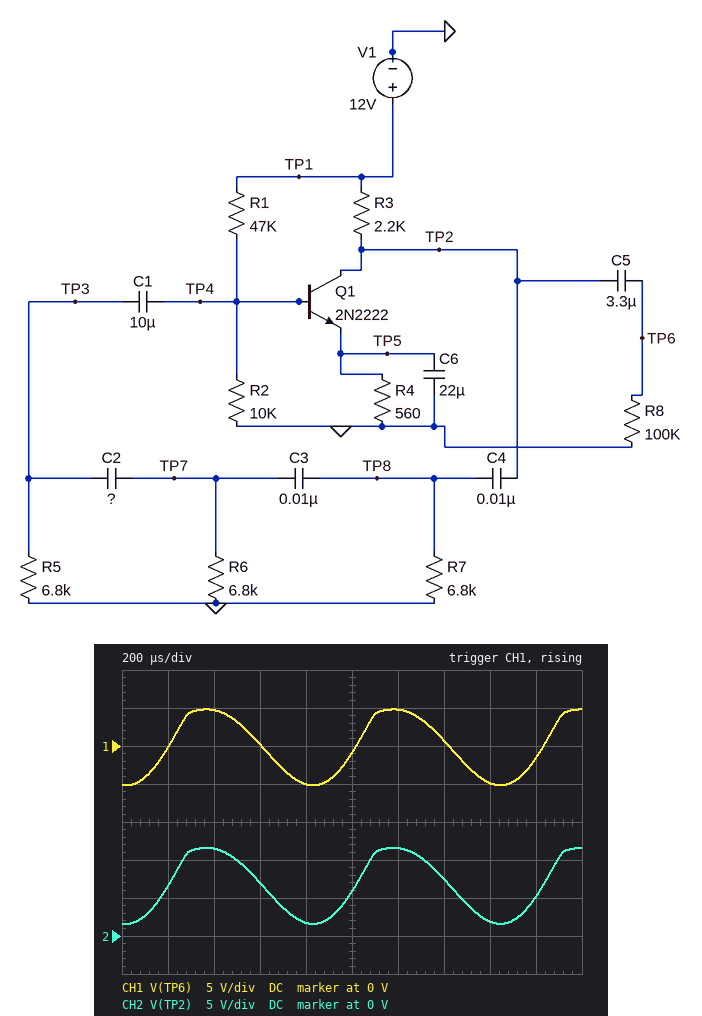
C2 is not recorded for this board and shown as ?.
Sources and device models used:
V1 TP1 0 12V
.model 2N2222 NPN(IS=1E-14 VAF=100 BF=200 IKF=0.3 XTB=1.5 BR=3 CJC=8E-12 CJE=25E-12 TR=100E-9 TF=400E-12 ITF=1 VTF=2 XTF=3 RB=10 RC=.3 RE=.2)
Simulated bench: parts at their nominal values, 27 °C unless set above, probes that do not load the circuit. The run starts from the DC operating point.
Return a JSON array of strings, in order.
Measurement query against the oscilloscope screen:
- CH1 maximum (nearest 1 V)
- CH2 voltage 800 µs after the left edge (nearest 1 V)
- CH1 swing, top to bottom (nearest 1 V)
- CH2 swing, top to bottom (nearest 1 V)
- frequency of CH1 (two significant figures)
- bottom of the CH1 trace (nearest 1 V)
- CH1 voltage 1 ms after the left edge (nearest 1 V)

["5 V", "2 V", "10 V", "10 V", "1.2 kHz", "-5 V", "-1 V"]
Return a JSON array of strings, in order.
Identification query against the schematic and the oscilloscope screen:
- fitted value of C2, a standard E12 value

["5.6 nF"]
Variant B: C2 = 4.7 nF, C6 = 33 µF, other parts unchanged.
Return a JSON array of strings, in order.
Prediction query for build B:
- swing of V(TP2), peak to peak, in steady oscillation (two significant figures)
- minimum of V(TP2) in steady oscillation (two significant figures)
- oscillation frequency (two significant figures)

["9.7 V", "1.8 V", "1.3 kHz"]
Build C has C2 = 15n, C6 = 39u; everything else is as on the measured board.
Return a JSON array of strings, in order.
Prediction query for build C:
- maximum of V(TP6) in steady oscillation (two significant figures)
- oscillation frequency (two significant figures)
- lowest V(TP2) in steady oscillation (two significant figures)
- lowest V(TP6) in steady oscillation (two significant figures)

["4.9 V", "890 Hz", "1.4 V", "-5.3 V"]
